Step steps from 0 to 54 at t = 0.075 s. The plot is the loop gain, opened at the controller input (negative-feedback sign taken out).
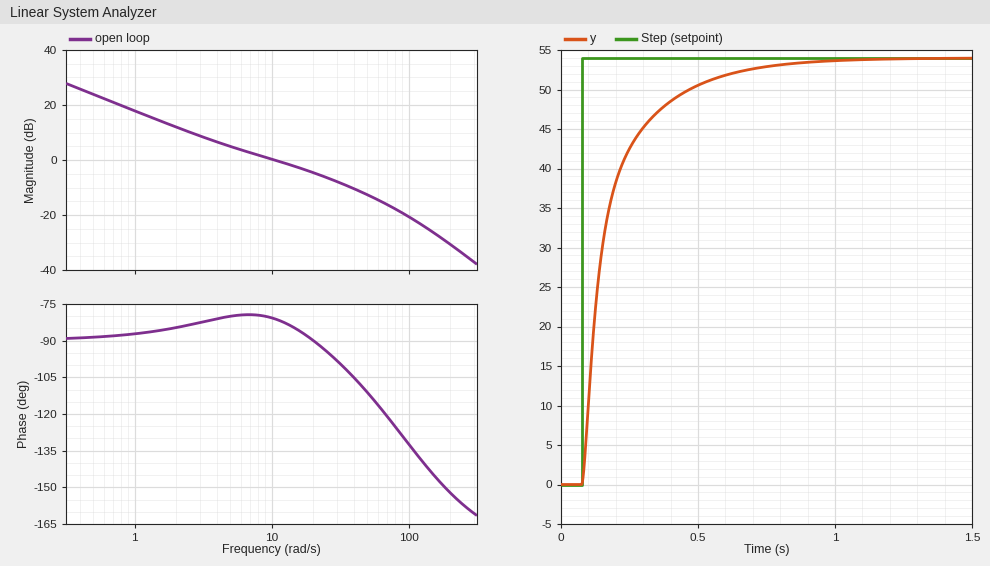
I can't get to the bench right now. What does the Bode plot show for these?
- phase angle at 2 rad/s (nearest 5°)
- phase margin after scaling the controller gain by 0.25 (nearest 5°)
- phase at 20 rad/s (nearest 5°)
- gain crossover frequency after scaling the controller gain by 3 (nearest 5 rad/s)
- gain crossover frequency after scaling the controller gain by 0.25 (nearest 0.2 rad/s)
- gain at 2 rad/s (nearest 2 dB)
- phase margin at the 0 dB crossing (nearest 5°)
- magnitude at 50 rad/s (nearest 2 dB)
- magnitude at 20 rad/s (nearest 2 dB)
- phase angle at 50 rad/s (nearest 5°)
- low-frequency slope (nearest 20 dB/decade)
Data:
-85°
95°
-90°
35 rad/s
2.0 rad/s
12 dB
100°
-12 dB
-4 dB
-110°
-20 dB/decade
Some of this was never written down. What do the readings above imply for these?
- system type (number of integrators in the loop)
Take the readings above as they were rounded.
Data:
1
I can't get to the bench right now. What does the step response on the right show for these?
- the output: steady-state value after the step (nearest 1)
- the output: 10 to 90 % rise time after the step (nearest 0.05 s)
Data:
54
0.30 s
